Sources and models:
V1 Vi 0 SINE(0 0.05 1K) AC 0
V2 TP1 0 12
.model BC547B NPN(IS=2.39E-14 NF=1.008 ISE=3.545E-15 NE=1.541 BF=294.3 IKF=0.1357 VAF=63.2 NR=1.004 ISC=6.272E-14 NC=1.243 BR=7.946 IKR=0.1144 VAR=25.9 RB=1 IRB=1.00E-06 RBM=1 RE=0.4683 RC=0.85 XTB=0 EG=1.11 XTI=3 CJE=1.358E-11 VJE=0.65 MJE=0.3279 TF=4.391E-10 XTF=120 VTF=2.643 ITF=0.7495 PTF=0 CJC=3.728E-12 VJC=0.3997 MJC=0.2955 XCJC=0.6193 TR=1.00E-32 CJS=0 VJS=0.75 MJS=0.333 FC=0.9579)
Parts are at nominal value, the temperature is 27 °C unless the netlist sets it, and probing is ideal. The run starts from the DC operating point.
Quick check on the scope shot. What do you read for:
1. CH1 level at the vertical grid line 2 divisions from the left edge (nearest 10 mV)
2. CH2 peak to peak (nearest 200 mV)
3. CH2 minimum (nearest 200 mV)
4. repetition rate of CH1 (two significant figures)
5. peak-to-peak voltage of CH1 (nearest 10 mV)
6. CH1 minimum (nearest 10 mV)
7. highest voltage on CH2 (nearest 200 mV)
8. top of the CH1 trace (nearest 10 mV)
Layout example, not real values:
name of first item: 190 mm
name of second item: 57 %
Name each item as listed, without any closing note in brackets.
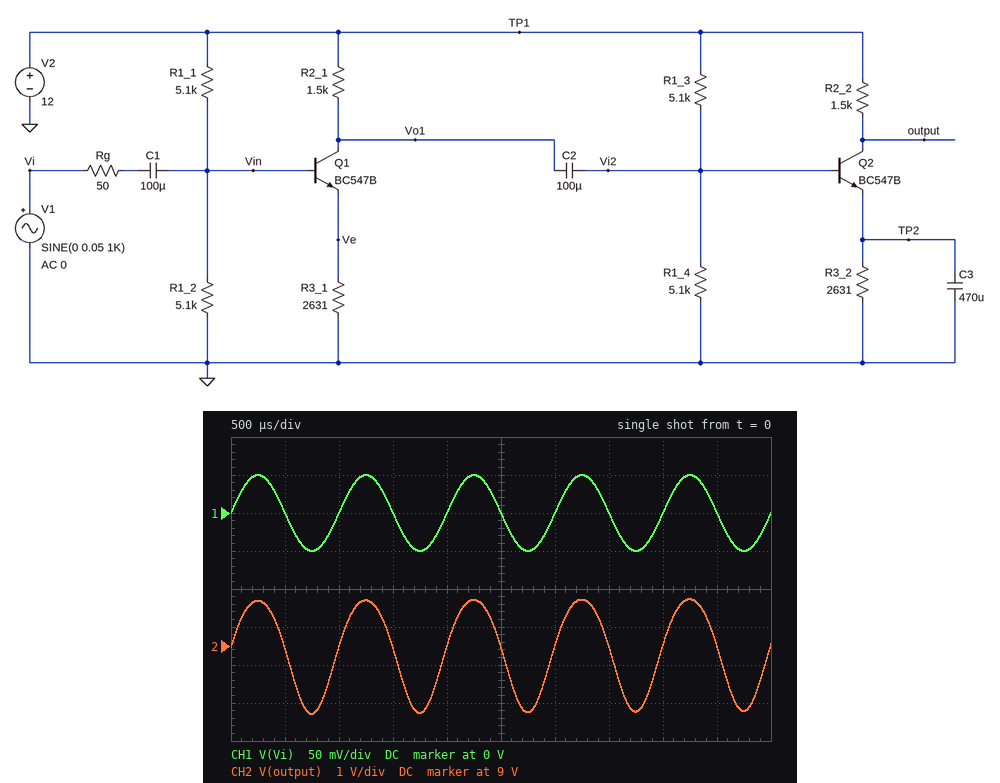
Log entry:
CH1 level at the vertical grid line 2 divisions from the left edge: 0 V
CH2 peak to peak: 3.0 V
CH2 minimum: 7.2 V
repetition rate of CH1: 1.0 kHz
peak-to-peak voltage of CH1: 100 mV
CH1 minimum: -50 mV
highest voltage on CH2: 10.2 V
top of the CH1 trace: 50 mV
